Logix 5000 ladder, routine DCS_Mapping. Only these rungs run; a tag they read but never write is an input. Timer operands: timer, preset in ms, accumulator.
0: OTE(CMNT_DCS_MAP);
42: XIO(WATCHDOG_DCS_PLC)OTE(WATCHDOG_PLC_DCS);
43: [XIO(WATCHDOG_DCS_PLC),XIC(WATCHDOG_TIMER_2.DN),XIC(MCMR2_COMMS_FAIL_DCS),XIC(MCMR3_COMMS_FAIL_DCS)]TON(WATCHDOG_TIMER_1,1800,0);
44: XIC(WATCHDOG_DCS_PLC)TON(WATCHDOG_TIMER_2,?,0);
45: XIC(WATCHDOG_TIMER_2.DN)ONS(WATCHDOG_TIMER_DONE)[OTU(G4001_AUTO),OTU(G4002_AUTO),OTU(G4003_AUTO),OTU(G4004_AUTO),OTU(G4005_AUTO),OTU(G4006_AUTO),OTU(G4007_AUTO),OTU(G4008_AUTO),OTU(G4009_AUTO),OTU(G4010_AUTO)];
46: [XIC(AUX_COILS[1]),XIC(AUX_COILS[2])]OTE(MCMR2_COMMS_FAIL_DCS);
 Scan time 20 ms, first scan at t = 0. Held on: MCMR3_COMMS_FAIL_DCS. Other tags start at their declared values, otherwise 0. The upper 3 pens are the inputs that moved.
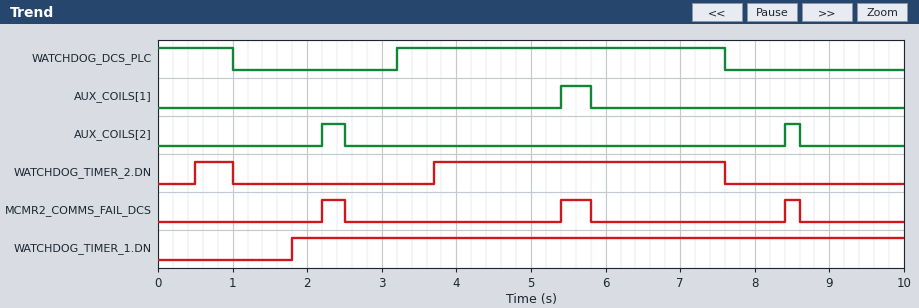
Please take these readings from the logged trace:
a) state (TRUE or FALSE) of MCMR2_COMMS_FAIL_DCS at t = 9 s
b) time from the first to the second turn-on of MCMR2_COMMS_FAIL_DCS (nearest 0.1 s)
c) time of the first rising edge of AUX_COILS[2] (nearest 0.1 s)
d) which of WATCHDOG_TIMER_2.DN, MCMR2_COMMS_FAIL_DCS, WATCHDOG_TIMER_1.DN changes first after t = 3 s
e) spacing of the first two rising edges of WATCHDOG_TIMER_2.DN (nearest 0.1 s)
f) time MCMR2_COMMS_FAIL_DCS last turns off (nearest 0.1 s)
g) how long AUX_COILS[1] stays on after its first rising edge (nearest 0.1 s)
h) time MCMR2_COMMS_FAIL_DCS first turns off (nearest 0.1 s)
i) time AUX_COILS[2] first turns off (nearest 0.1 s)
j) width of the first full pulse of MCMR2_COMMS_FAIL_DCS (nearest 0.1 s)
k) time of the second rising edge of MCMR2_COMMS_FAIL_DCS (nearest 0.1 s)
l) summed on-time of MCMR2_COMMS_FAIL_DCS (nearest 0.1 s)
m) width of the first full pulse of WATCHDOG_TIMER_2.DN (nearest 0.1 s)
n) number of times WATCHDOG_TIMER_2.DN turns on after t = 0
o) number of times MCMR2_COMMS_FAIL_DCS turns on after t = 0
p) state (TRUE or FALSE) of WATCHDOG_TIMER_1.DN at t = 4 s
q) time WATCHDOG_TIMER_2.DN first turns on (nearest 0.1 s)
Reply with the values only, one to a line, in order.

FALSE
3.2 s
2.2 s
WATCHDOG_TIMER_2.DN
3.2 s
8.6 s
0.4 s
2.5 s
2.5 s
0.3 s
5.4 s
0.9 s
0.5 s
2
3
TRUE
0.5 s
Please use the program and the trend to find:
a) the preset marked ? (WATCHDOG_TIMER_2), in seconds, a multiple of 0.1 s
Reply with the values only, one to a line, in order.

0.5 s
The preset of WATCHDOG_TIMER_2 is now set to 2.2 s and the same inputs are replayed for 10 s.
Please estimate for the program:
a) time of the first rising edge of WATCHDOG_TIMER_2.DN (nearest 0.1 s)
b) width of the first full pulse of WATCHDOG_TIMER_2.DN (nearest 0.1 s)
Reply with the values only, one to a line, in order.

5.4 s
2.2 s
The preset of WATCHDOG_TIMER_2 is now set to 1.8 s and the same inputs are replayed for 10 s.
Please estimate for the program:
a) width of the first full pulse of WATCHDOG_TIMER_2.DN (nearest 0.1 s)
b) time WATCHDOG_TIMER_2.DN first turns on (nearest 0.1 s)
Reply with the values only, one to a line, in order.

2.6 s
5.0 s
